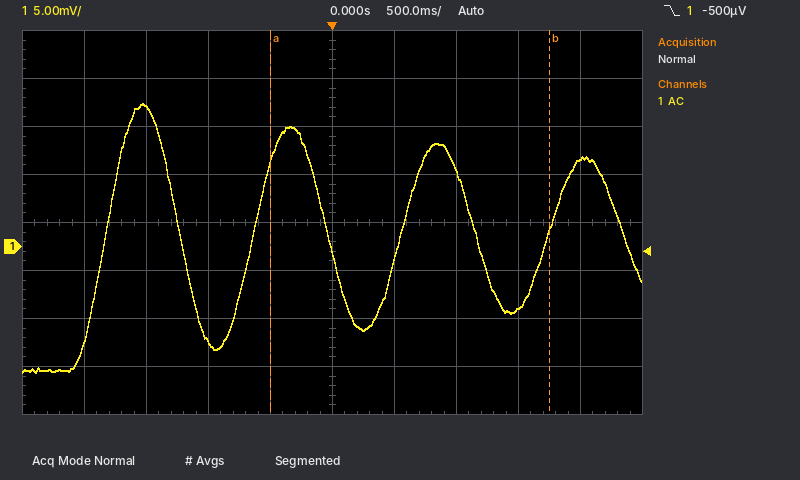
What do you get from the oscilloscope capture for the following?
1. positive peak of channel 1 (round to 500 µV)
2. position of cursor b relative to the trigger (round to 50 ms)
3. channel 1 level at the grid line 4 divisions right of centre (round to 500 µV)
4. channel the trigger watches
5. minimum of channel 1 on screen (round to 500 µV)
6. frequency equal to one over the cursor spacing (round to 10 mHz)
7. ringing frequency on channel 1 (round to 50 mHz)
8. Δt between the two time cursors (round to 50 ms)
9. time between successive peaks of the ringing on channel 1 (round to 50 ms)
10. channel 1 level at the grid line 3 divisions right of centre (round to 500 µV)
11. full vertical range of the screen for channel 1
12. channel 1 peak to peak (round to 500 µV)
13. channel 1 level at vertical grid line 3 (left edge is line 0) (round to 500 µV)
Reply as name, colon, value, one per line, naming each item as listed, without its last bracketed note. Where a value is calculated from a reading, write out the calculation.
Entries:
positive peak of channel 1: 15.0 mV
position of cursor b relative to the trigger: +1.75 s
channel 1 level at the grid line 4 divisions right of centre: 9.0 mV
channel the trigger watches: channel 1
minimum of channel 1 on screen: -13.0 mV
frequency equal to one over the cursor spacing: 1 / 2.25 s ≈ 440 mHz
ringing frequency on channel 1: 1 / 1.20 s ≈ 833 mHz, so 850 mHz to the nearest 50 mHz
Δt between the two time cursors: 2.25 s
time between successive peaks of the ringing on channel 1: 1.20 s
channel 1 level at the grid line 3 divisions right of centre: -6.5 mV
full vertical range of the screen for channel 1: 40 mV
channel 1 peak to peak: 15.0 mV − (-13.0 mV) = 28.0 mV
channel 1 level at vertical grid line 3 (left edge is line 0): -10.0 mV
